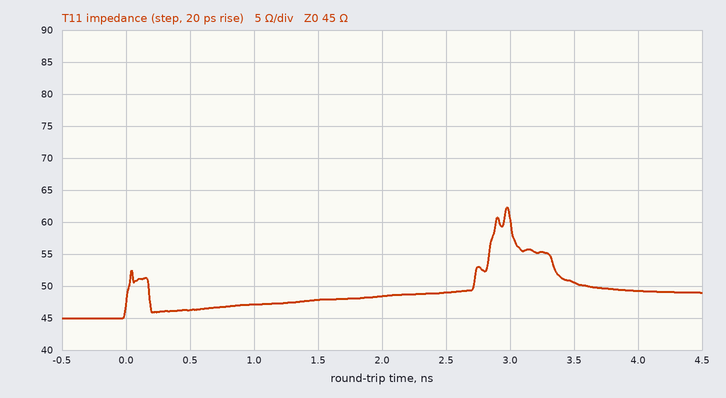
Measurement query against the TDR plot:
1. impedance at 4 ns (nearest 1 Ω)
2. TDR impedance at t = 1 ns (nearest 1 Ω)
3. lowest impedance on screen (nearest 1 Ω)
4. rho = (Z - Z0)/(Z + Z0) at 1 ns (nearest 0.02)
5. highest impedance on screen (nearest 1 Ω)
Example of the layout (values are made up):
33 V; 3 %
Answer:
49 Ω; 47 Ω; 45 Ω; +0.02; 62 Ω
